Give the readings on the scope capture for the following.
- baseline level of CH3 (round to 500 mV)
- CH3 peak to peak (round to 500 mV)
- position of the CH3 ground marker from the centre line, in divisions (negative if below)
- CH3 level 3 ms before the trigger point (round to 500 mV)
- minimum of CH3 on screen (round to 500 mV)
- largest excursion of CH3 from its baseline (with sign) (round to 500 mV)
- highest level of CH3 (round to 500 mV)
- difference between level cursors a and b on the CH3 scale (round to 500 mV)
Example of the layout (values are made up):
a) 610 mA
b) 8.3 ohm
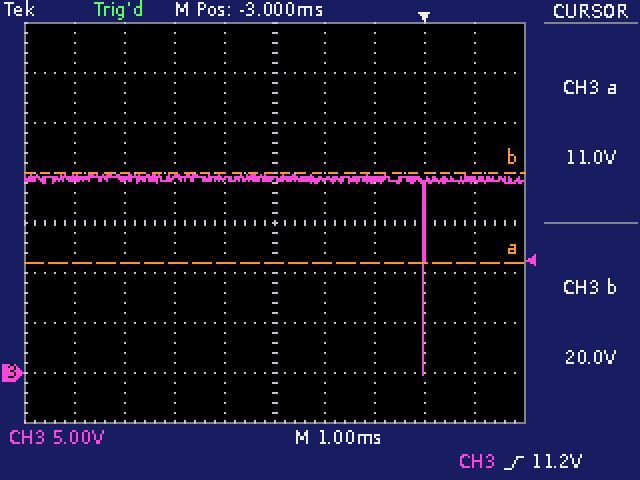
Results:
a) 19.5 V
b) 20.0 V
c) -3.0 div
d) 19.5 V
e) 0.0 V
f) -19.5 V
g) 20.0 V
h) 9.0 V
